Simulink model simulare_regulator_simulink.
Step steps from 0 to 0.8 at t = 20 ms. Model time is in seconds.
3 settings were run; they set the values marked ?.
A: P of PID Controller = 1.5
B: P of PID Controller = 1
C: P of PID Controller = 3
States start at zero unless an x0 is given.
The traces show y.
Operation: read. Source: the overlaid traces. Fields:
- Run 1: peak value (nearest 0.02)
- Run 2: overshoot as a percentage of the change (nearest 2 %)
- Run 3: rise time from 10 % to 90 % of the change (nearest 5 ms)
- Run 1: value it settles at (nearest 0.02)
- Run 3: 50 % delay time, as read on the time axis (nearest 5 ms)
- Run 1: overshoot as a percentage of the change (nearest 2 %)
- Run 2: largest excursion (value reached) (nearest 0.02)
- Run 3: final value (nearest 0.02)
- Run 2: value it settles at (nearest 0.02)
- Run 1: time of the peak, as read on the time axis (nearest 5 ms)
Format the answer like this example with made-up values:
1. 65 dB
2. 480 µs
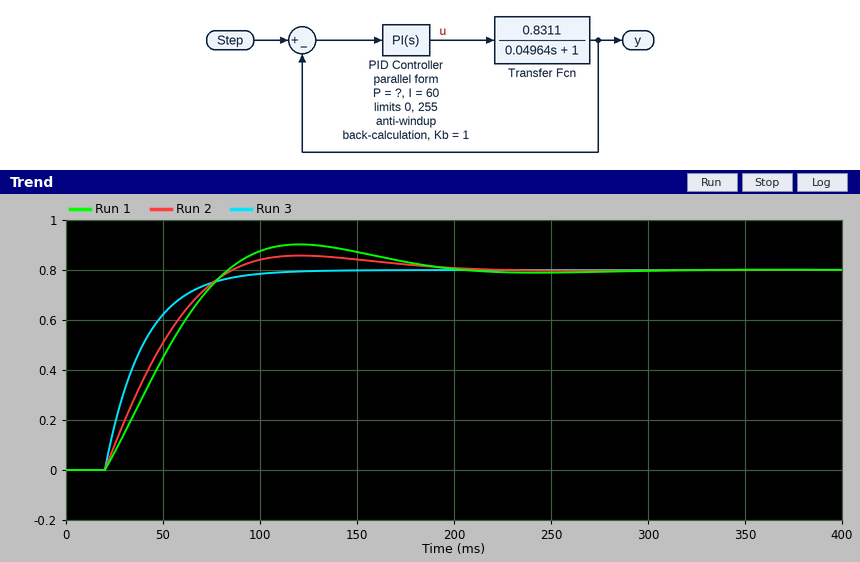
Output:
1. 0.90
2. 8 %
3. 45 ms
4. 0.80
5. 35 ms
6. 12 %
7. 0.86
8. 0.80
9. 0.80
10. 120 ms
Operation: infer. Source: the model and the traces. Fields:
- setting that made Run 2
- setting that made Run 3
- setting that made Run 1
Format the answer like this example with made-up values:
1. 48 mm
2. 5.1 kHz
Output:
1. A
2. C
3. B
